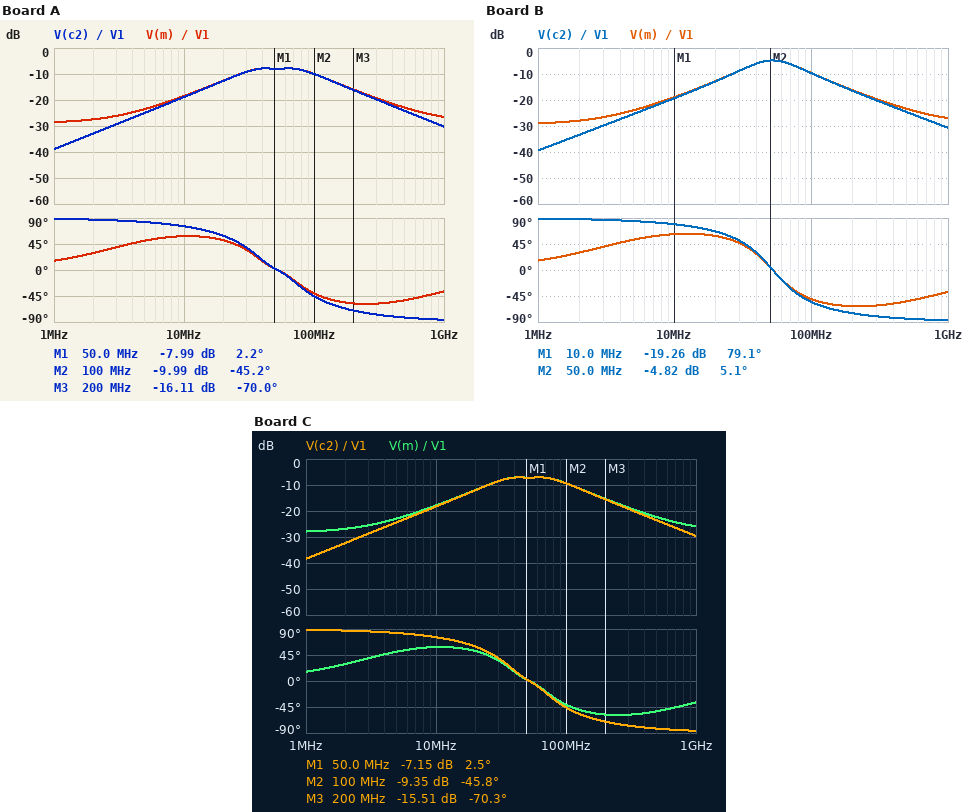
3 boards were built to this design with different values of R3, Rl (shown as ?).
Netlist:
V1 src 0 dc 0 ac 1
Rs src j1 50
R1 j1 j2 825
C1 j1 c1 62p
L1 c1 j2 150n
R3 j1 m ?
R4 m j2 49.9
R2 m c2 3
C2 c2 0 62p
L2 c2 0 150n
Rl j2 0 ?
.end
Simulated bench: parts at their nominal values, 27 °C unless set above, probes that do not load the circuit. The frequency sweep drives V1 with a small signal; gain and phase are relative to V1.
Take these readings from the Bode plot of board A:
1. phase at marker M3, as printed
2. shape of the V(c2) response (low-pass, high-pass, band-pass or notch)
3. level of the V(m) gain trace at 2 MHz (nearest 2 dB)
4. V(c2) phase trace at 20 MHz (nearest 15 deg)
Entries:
-70.0 deg
band-pass
-28 dB
60 deg
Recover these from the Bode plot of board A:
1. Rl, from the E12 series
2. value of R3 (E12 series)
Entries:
33 Ω
27 Ω
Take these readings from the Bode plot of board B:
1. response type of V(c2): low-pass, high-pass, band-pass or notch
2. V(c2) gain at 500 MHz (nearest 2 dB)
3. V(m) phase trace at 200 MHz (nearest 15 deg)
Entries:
band-pass
-24 dB
-60 deg
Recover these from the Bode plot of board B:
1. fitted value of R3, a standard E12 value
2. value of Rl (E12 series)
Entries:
33 Ω
68 Ω
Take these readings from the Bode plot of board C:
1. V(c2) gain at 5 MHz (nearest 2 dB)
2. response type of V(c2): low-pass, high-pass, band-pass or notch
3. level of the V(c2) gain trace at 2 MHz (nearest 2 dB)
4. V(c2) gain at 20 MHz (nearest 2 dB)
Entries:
-24 dB
band-pass
-32 dB
-12 dB
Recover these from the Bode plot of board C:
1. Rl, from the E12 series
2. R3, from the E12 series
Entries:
39 Ω
22 Ω
